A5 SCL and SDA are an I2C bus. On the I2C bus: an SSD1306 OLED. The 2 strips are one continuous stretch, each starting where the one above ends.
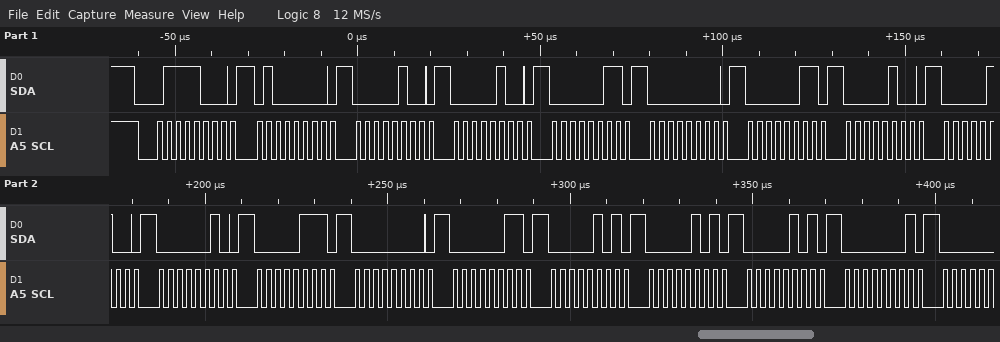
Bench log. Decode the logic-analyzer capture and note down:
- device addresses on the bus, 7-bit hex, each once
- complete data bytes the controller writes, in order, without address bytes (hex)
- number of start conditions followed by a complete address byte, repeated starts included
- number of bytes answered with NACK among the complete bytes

0x3C
40 04 04 03 00 03 04 04 02 07 00 03 05 05 05 01
1
0
